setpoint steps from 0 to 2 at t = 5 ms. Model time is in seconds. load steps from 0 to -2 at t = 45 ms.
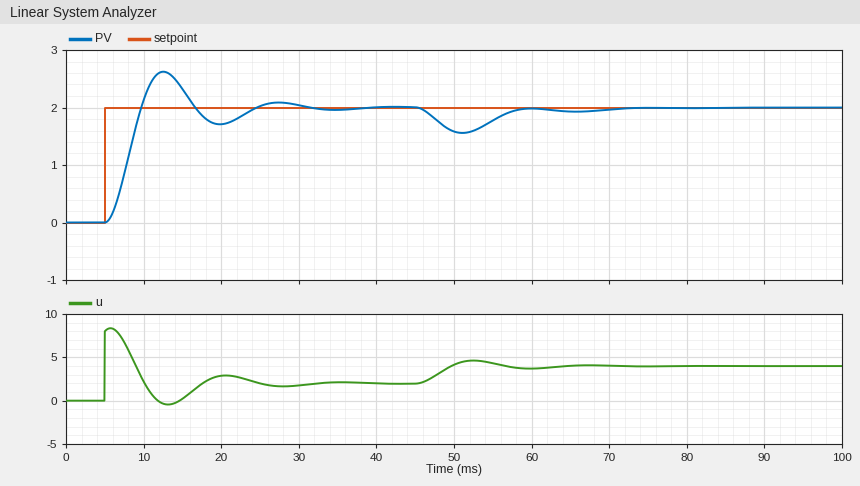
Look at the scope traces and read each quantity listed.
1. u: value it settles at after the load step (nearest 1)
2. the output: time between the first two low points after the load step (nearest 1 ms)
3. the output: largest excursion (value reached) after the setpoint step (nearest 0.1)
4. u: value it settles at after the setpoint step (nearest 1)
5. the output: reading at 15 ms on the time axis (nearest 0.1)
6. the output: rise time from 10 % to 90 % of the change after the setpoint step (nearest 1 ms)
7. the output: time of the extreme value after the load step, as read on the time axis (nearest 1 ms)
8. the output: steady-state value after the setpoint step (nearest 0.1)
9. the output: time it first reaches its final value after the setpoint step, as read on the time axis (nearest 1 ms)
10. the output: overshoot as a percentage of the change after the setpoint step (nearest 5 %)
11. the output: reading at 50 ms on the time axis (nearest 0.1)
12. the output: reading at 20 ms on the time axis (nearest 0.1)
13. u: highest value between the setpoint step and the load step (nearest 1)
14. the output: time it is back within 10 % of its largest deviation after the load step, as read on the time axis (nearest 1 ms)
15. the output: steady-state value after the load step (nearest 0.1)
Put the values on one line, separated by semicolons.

4; 15 ms; 2.6; 2; 2.3; 3 ms; 51 ms; 2.0; 10 ms; 30 %; 1.6; 1.7; 8; 69 ms; 2.0
